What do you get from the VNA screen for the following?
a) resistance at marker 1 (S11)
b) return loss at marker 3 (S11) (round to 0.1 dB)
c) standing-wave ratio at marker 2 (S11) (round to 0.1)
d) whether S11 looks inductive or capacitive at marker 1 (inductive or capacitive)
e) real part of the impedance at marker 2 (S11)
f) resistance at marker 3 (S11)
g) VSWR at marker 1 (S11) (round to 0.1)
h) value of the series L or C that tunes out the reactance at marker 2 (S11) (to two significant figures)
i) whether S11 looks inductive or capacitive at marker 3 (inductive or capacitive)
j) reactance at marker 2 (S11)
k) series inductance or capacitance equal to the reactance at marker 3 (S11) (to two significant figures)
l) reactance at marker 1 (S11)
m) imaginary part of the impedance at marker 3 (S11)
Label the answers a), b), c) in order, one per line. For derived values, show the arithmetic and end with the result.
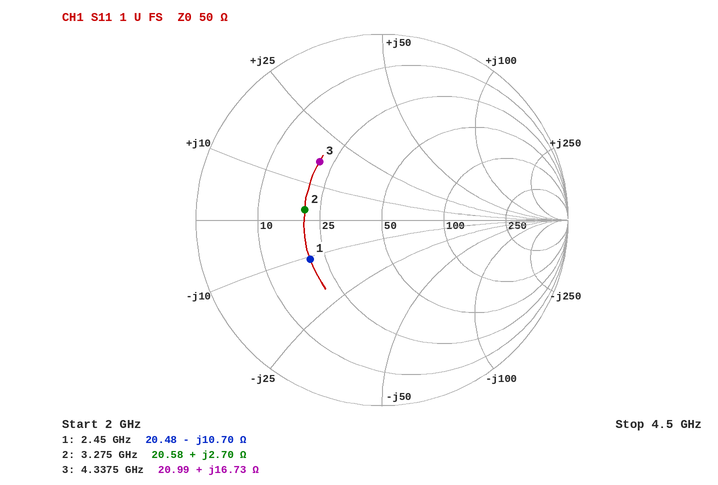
a) 20.48 Ω
b) 6.8 dB
c) 2.4
d) capacitive
e) 20.58 Ω
f) 20.99 Ω
g) 2.6
h) C = 1/(2π × 3.275 GHz × 2.7 Ω) ≈ 18 pF
i) inductive
j) +2.70 Ω
k) L = 16.73 Ω/(2π × 4.3375 GHz) ≈ 614 pH, so 610 pH to two significant figures
l) -10.70 Ω
m) +16.73 Ω
